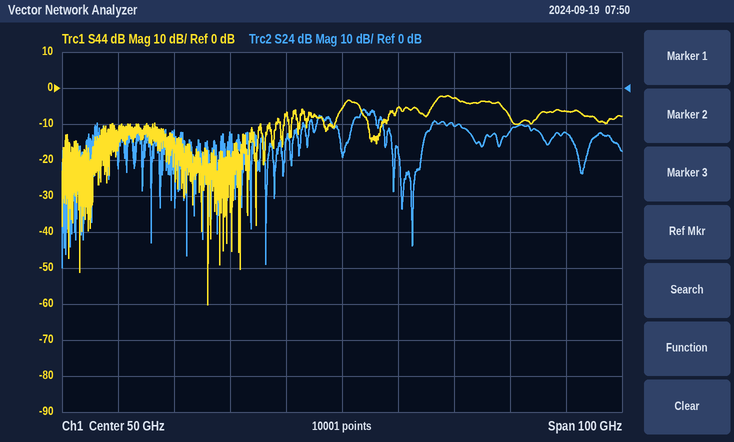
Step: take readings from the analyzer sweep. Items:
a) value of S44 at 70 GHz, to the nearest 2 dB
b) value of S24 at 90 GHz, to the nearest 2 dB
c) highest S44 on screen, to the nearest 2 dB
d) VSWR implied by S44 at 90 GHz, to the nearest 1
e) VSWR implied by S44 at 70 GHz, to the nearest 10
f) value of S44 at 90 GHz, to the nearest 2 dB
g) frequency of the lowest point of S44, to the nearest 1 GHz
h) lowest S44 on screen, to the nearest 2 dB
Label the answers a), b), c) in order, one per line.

a) -2 dB
b) -12 dB
c) -2 dB
d) 3
e) 10
f) -6 dB
g) 26 GHz
h) -60 dB
